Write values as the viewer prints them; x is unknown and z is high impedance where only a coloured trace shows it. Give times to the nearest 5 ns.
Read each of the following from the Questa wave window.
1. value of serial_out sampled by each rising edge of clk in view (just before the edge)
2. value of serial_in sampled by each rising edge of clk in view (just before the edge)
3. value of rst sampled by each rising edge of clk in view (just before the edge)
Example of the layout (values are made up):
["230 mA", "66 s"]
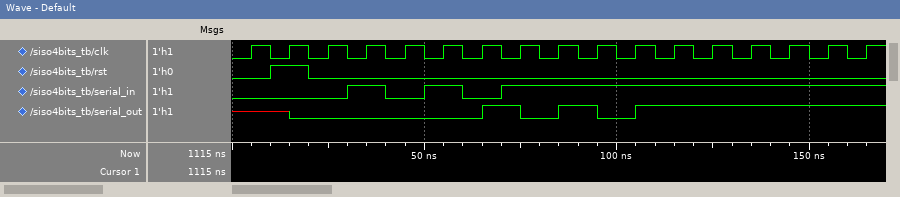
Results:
["x x 0 0 0 0 0 1 0 1 0 1 1 1 1 1 1", "0 0 0 1 0 1 0 1 1 1 1 1 1 1 1 1 1", "0 1 0 0 0 0 0 0 0 0 0 0 0 0 0 0 0"]
